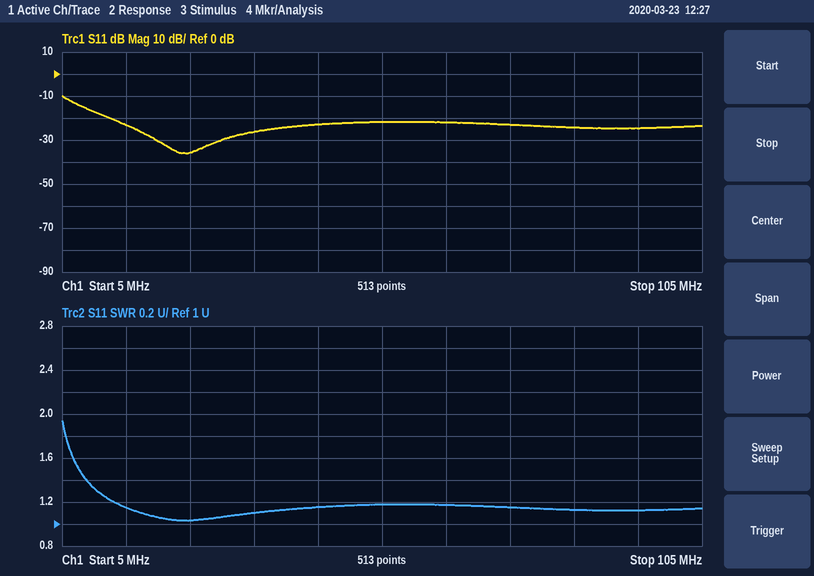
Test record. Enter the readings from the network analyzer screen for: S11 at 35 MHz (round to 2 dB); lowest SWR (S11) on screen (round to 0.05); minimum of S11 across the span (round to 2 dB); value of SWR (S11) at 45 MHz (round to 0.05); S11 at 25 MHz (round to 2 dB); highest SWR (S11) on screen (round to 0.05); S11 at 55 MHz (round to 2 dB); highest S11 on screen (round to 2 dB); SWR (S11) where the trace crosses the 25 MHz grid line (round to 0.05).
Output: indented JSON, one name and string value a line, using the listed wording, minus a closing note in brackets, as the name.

{
  "S11 at 35 MHz": "-26 dB",
  "lowest SWR (S11) on screen": "1.05",
  "minimum of S11 across the span": "-36 dB",
  "value of SWR (S11) at 45 MHz": "1.15",
  "S11 at 25 MHz": "-36 dB",
  "highest SWR (S11) on screen": "1.95",
  "S11 at 55 MHz": "-22 dB",
  "highest S11 on screen": "-10 dB",
  "SWR (S11) where the trace crosses the 25 MHz grid line": "1.05"
}
